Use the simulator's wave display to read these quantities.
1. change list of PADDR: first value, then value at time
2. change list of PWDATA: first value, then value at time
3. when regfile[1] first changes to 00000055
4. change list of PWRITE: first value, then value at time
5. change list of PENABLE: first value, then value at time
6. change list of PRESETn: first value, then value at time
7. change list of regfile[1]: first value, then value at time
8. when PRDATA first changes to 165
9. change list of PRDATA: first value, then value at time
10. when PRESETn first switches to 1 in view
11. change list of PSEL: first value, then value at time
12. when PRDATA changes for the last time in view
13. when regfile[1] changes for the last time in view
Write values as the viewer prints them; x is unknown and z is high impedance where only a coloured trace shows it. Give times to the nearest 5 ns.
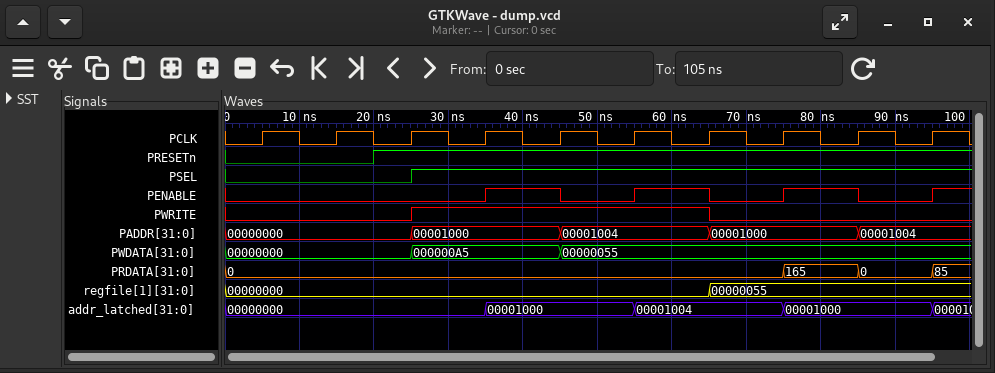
00000000, 00001000 at 25 ns, 00001004 at 45 ns, 00001000 at 65 ns, 00001004 at 85 ns
00000000, 000000A5 at 25 ns, 00000055 at 45 ns
65 ns
0, 1 at 25 ns, 0 at 65 ns
0, 1 at 35 ns, 0 at 45 ns, 1 at 55 ns, 0 at 65 ns, 1 at 75 ns, 0 at 85 ns, 1 at 95 ns
0, 1 at 20 ns
00000000, 00000055 at 65 ns
75 ns
0, 165 at 75 ns, 0 at 85 ns, 85 at 95 ns
20 ns
0, 1 at 25 ns
95 ns
65 ns
